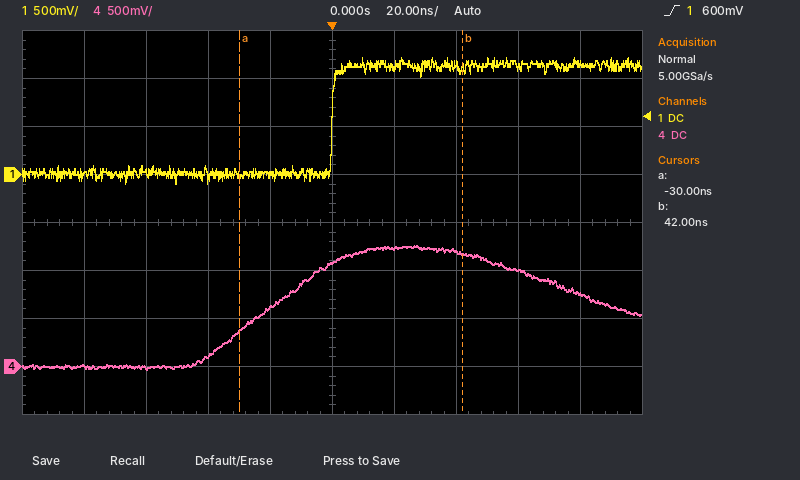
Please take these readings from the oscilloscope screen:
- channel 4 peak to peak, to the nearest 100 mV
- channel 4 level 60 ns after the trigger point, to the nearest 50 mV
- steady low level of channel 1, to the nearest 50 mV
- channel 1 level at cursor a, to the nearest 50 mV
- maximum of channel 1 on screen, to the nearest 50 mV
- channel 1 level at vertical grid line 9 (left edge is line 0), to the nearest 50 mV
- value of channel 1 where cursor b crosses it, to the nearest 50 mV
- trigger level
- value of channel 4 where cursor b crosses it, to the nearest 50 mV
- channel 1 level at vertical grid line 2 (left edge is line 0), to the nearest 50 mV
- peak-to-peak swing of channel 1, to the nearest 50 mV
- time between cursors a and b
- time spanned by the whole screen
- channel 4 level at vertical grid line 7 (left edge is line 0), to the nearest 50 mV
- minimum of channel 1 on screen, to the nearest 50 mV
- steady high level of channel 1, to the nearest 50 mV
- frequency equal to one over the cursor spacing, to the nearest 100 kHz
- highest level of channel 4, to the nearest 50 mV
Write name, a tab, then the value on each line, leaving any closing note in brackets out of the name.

channel 4 peak to peak, to the nearest 100 mV	1.30 V
channel 4 level 60 ns after the trigger point, to the nearest 50 mV	1.00 V
steady low level of channel 1, to the nearest 50 mV	0 mV
channel 1 level at cursor a, to the nearest 50 mV	0 mV
maximum of channel 1 on screen, to the nearest 50 mV	1.20 V
channel 1 level at vertical grid line 9 (left edge is line 0), to the nearest 50 mV	1.15 V
value of channel 1 where cursor b crosses it, to the nearest 50 mV	1.10 V
trigger level	600 mV
value of channel 4 where cursor b crosses it, to the nearest 50 mV	1.20 V
channel 1 level at vertical grid line 2 (left edge is line 0), to the nearest 50 mV	0 mV
peak-to-peak swing of channel 1, to the nearest 50 mV	1.30 V
time between cursors a and b	72 ns
time spanned by the whole screen	200 ns
channel 4 level at vertical grid line 7 (left edge is line 0), to the nearest 50 mV	1.20 V
minimum of channel 1 on screen, to the nearest 50 mV	-100 mV
steady high level of channel 1, to the nearest 50 mV	1.15 V
frequency equal to one over the cursor spacing, to the nearest 100 kHz	13.9 MHz
highest level of channel 4, to the nearest 50 mV	1.25 V
